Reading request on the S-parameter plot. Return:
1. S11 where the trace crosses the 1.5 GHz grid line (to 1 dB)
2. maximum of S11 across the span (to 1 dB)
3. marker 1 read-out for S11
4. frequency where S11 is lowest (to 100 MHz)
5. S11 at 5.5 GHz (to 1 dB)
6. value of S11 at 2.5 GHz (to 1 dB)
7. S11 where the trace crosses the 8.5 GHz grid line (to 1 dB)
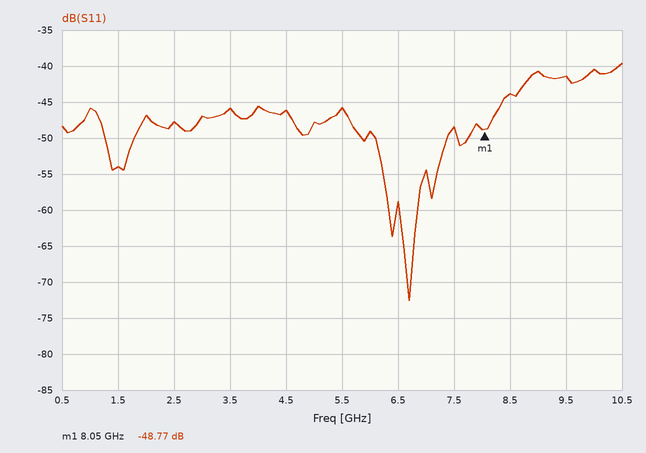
-54 dB
-40 dB
-48.77 dB
6.7 GHz
-46 dB
-48 dB
-44 dB
